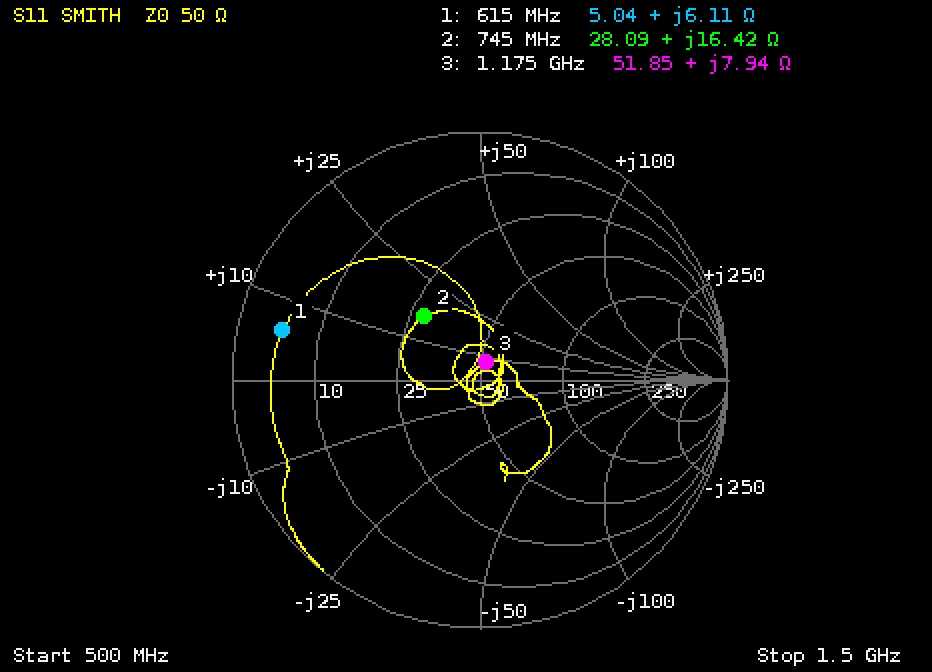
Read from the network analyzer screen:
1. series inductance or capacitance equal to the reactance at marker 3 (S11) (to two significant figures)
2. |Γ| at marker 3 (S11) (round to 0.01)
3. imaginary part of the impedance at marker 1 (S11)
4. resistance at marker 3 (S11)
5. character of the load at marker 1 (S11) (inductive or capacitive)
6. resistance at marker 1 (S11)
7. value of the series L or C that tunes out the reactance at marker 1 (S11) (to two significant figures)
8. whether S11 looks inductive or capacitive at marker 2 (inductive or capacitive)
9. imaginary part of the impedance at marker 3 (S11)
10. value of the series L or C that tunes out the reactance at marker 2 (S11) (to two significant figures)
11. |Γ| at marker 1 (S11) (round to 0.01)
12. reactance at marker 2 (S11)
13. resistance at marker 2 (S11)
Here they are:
1.1 nH
0.08
+6.11 Ω
51.85 Ω
inductive
5.04 Ω
42 pF
inductive
+7.94 Ω
13 pF
0.82
+16.42 Ω
28.09 Ω
